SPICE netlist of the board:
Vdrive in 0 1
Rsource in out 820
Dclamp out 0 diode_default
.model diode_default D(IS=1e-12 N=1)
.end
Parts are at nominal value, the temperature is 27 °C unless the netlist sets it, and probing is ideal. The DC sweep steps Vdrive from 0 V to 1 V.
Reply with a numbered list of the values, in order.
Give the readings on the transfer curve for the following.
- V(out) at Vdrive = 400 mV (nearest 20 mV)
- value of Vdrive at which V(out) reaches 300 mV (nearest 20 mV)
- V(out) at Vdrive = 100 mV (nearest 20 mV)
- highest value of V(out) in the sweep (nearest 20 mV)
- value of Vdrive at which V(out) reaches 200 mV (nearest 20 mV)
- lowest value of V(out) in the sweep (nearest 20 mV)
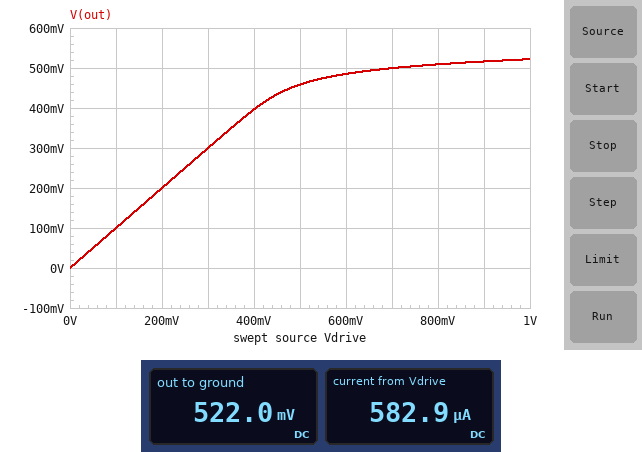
1. 400 mV
2. 300 mV
3. 100 mV
4. 520 mV
5. 200 mV
6. 0 V
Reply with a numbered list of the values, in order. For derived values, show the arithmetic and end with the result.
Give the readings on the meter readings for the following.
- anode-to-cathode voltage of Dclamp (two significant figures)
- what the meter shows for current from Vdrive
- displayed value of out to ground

1. 522 mV = 520 mV
2. 582.9 µA
3. 522.0 mV
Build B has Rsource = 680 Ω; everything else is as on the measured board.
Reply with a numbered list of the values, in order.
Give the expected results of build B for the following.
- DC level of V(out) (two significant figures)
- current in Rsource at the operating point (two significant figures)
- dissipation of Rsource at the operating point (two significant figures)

1. 530 mV
2. 700 µA
3. 330 µW
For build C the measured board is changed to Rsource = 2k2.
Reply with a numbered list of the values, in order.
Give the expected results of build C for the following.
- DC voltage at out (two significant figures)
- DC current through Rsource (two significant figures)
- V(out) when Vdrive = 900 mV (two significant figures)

1. 500 mV
2. 230 µA
3. 490 mV
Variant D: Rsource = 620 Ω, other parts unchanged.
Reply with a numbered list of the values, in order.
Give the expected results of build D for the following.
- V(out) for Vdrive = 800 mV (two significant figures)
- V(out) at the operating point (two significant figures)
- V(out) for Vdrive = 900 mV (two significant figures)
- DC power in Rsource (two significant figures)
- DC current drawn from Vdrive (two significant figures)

1. 520 mV
2. 530 mV
3. 520 mV
4. 360 µW
5. 760 µA
